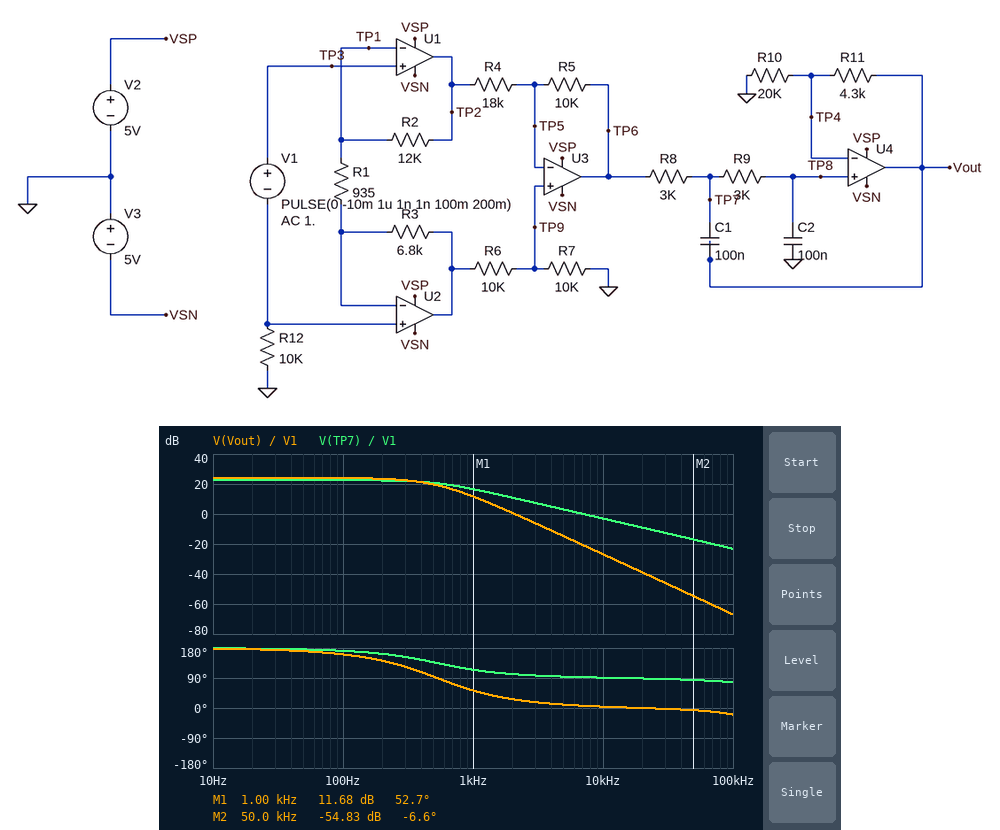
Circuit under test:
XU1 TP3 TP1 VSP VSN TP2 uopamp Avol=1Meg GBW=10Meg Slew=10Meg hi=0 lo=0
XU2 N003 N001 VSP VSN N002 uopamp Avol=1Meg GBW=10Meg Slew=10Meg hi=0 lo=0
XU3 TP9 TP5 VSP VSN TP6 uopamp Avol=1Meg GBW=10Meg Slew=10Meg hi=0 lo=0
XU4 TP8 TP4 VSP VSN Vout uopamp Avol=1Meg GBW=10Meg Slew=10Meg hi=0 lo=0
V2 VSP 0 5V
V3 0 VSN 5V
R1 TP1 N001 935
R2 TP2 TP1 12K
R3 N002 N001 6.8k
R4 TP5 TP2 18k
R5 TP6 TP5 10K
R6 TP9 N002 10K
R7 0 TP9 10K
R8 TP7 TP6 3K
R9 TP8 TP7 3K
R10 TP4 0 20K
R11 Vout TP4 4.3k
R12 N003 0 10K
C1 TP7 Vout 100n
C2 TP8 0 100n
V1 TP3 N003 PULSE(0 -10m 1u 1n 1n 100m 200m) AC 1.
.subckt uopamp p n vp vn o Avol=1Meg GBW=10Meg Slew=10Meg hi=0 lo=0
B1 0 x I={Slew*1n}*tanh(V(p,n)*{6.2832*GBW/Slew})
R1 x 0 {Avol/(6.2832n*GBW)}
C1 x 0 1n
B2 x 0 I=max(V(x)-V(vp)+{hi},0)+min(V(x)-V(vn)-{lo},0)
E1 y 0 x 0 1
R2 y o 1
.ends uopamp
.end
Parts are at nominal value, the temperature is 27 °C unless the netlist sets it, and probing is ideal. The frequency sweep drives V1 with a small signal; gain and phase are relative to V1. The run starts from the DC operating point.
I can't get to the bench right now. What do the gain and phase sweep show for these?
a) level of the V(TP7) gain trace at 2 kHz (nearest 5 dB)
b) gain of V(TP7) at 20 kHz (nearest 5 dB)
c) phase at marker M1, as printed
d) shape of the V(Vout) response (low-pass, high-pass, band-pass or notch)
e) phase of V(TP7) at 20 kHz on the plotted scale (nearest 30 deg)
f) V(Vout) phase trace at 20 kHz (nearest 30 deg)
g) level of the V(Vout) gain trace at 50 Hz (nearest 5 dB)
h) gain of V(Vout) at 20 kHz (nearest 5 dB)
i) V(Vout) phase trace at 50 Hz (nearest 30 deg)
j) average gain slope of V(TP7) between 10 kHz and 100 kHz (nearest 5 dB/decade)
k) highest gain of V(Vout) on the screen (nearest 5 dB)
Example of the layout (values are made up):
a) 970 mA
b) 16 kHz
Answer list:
a) 10 dB
b) -10 dB
c) 52.7 deg
d) low-pass
e) 90 deg
f) 0 deg
g) 25 dB
h) -40 dB
i) 180 deg
j) -20 dB/decade
k) 25 dB
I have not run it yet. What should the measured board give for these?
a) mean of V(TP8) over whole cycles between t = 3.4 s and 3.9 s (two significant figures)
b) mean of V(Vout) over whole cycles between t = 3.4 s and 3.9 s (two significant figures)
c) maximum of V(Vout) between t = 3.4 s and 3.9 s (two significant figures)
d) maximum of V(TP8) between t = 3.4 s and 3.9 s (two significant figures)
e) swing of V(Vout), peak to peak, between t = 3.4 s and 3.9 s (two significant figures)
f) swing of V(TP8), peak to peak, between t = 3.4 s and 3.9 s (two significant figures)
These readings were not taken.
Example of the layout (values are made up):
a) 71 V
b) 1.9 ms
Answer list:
a) 67 mV
b) 81 mV
c) 160 mV
d) 130 mV
e) 160 mV
f) 130 mV
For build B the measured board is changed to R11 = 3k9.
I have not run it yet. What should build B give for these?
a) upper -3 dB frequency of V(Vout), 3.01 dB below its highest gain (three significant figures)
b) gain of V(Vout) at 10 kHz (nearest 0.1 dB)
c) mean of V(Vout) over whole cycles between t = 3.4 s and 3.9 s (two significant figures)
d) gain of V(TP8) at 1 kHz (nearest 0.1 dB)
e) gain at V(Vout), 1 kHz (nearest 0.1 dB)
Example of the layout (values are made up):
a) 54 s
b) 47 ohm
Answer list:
a) 394 Hz
b) -27.0 dB
c) 80 mV
d) 9.9 dB
e) 11.5 dB
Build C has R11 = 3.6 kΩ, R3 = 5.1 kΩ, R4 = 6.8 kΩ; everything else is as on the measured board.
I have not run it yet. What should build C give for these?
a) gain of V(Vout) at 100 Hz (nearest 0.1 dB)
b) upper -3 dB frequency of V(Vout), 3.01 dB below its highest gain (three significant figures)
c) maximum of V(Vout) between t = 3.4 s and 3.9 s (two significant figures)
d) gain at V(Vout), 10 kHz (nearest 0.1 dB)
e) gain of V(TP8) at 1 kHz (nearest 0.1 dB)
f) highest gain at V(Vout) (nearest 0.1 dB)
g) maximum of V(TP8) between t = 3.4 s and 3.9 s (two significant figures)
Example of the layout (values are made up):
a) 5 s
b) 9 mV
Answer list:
a) 29.9 dB
b) 390 Hz
c) 320 mV
d) -20.9 dB
e) 16.0 dB
f) 30.1 dB
g) 270 mV
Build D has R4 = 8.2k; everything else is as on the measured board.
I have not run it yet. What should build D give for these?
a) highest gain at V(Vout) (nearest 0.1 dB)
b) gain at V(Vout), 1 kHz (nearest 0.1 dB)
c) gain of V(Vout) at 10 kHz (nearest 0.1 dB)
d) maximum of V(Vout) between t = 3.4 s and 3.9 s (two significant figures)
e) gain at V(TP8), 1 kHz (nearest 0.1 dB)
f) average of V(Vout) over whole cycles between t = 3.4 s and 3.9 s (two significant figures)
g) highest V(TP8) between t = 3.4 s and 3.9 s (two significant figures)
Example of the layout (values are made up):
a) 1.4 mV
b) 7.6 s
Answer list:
a) 29.6 dB
b) 17.1 dB
c) -21.4 dB
d) 300 mV
e) 15.4 dB
f) 150 mV
g) 250 mV
